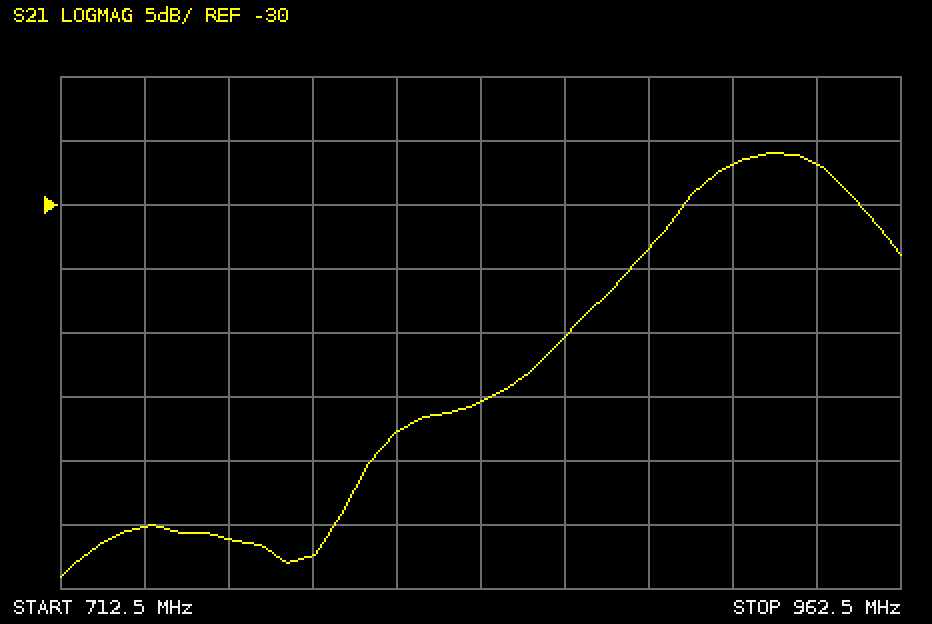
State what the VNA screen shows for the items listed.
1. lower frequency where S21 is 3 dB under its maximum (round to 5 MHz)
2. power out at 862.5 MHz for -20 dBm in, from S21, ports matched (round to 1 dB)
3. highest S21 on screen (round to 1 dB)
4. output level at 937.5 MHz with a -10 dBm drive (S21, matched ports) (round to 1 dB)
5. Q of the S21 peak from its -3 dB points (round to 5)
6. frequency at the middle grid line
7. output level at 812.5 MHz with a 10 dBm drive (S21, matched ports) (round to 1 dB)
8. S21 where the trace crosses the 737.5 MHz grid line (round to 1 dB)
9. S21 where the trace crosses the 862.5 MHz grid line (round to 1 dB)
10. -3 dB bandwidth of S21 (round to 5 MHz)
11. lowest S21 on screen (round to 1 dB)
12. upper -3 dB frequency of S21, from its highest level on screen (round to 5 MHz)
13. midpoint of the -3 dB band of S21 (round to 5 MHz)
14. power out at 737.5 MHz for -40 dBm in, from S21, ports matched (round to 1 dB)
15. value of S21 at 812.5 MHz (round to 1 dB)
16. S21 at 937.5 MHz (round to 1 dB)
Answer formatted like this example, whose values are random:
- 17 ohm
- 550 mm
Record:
- 900 MHz
- -60 dBm
- -26 dB
- -37 dBm
- 20
- 837.5 MHz
- -38 dBm
- -55 dB
- -40 dB
- 45 MHz
- -59 dB
- 945 MHz
- 925 MHz
- -95 dBm
- -48 dB
- -27 dB
